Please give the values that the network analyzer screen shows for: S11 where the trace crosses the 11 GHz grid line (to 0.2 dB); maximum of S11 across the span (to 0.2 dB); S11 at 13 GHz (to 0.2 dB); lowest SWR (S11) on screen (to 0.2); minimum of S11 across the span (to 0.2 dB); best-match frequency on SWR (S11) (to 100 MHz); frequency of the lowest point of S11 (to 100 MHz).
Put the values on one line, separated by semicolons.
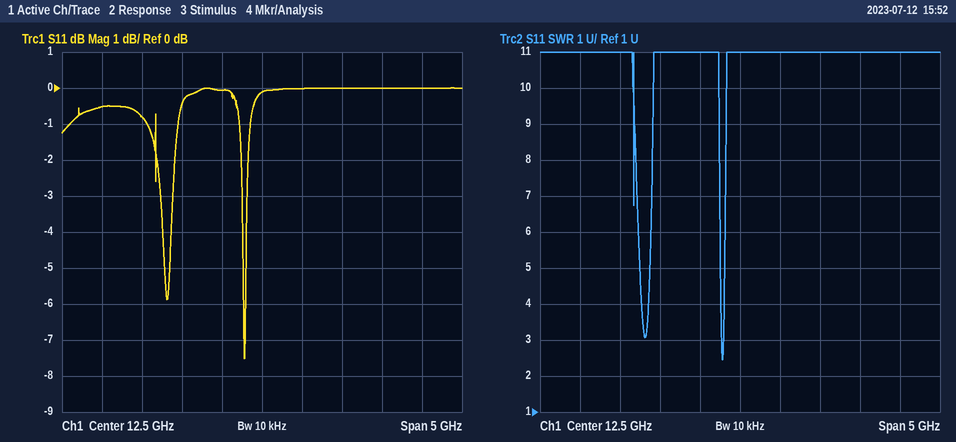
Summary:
-0.8 dB; 0.0 dB; 0.0 dB; 2.4; -7.6 dB; 12.3 GHz; 12.3 GHz
